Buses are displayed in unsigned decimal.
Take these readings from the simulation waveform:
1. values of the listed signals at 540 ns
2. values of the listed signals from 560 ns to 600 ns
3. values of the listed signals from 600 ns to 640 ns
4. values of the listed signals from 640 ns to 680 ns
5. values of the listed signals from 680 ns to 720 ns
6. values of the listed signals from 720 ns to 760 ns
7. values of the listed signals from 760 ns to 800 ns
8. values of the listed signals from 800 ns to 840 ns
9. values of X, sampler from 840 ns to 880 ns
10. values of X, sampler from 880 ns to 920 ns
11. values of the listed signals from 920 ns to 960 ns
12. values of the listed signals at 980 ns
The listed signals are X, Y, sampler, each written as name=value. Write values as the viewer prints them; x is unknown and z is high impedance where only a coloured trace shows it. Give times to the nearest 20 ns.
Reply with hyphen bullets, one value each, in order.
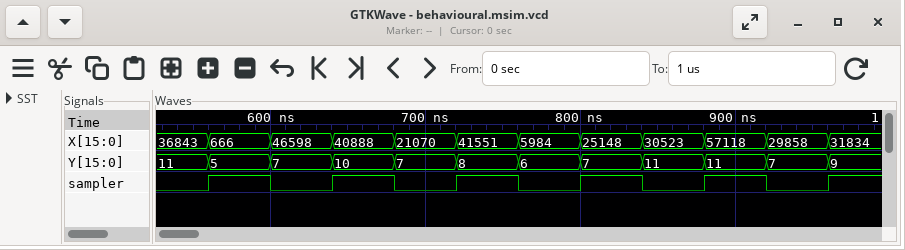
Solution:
- X=36843, Y=11, sampler=0
- X=666, Y=5, sampler=1
- X=46598, Y=7, sampler=0
- X=40888, Y=10, sampler=1
- X=21070, Y=7, sampler=0
- X=41551, Y=8, sampler=1
- X=5984, Y=6, sampler=0
- X=25148, Y=7, sampler=1
- X=30523, sampler=0
- X=57118, sampler=1
- X=29858, Y=7, sampler=0
- X=31834, Y=9, sampler=1
